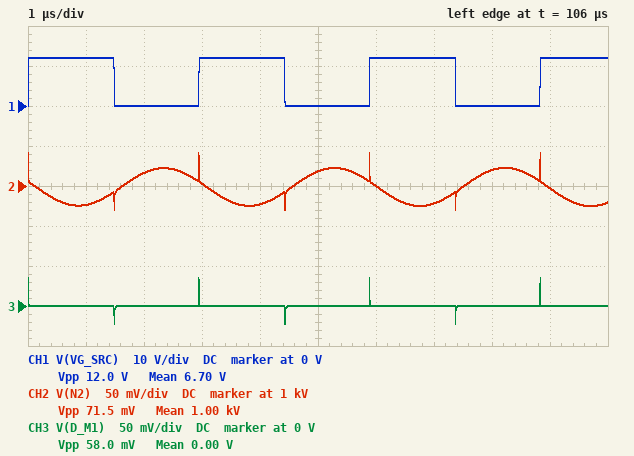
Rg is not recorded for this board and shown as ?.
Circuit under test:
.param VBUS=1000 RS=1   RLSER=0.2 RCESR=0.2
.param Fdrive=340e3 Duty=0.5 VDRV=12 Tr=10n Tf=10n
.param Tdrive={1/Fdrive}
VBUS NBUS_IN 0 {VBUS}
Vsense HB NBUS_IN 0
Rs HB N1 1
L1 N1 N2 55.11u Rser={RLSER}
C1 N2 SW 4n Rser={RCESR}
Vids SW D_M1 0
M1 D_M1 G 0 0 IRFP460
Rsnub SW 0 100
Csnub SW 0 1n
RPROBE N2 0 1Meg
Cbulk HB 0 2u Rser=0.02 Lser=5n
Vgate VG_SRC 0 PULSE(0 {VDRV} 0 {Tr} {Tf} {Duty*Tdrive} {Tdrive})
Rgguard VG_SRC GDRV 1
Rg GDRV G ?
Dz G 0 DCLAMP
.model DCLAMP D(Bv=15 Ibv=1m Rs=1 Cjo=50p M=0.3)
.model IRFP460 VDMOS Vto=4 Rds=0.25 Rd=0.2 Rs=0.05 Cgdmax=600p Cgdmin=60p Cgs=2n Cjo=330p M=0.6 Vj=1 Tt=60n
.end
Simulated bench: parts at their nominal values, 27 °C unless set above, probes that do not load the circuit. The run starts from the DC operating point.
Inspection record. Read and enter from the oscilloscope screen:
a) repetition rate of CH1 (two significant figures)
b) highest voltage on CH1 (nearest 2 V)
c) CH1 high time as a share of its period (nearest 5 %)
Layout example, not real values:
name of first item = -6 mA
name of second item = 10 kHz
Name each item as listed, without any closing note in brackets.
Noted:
repetition rate of CH1 = 340 kHz
highest voltage on CH1 = 12 V
CH1 high time as a share of its period = 50 %
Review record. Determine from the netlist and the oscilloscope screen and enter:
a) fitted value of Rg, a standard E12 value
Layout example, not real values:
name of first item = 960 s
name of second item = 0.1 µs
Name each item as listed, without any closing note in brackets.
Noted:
fitted value of Rg, a standard E12 value = 5.6 Ω
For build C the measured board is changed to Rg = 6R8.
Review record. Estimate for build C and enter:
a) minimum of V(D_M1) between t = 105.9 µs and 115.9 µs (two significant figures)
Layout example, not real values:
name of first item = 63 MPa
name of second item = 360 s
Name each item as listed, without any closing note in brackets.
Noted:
minimum of V(D_M1) between t = 105.9 µs and 115.9 µs = -20 mV
